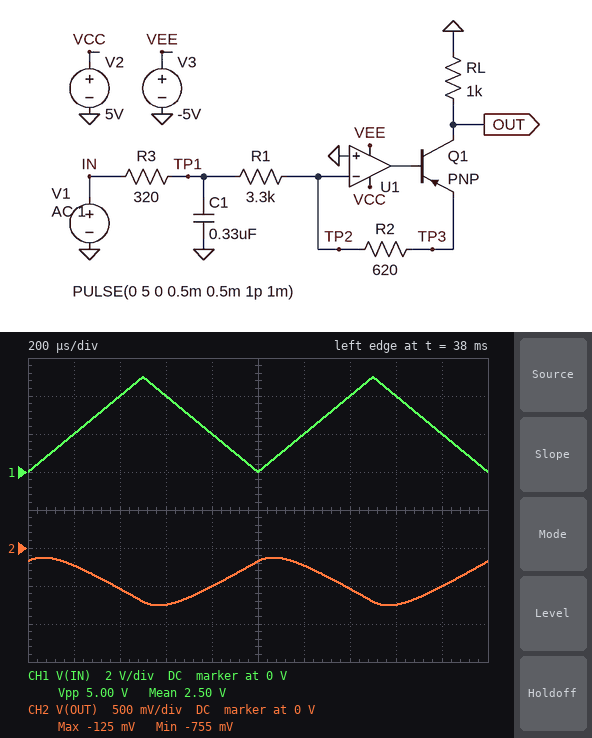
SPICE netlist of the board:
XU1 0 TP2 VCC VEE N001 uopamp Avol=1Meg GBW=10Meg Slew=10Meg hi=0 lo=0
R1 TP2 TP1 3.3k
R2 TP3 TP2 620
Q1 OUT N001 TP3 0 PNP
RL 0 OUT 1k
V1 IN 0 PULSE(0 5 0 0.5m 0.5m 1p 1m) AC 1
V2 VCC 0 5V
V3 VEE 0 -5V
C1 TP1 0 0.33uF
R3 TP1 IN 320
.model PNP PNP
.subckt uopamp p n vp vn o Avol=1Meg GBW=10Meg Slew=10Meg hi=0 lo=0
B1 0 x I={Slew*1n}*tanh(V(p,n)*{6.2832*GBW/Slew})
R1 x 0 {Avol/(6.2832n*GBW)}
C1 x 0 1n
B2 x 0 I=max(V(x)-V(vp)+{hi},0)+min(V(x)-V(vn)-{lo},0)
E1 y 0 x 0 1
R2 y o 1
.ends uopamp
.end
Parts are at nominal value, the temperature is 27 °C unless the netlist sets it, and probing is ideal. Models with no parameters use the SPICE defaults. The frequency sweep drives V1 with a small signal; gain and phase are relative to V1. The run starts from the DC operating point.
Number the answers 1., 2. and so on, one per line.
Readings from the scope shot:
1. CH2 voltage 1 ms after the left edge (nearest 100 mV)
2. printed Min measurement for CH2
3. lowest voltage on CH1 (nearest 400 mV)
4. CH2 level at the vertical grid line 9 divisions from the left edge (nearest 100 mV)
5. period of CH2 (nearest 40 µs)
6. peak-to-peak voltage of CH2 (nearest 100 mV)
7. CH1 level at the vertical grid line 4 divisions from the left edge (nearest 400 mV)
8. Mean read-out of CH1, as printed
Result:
1. -200 mV
2. -755 mV
3. 0 V
4. -500 mV
5. 1.00 ms
6. 600 mV
7. 2.0 V
8. 2.50 V
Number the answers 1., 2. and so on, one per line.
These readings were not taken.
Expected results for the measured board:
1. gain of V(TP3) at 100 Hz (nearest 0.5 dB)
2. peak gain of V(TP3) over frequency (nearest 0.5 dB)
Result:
1. 0 dB
2. 0 dB
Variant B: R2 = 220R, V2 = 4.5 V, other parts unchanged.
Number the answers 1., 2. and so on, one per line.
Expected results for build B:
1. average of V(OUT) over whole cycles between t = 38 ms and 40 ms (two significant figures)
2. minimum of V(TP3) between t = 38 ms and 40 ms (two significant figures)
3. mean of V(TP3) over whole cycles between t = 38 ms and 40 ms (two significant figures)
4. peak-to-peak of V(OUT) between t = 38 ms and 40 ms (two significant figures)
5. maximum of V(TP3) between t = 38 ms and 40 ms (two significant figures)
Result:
1. -170 mV
2. -260 mV
3. -150 mV
4. 220 mV
5. -40 mV
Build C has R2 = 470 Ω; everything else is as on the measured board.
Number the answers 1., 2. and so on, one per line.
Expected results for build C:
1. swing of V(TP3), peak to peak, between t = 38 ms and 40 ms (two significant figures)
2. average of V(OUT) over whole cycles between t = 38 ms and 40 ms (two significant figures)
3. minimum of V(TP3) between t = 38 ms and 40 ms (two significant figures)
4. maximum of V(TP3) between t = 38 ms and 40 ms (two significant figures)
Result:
1. 480 mV
2. -340 mV
3. -560 mV
4. -86 mV
